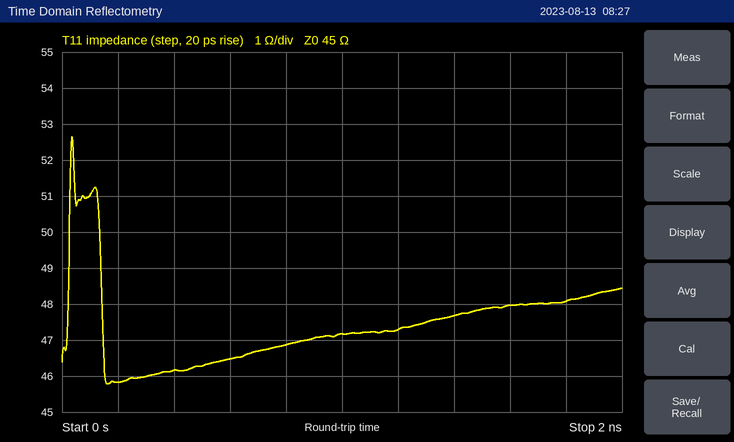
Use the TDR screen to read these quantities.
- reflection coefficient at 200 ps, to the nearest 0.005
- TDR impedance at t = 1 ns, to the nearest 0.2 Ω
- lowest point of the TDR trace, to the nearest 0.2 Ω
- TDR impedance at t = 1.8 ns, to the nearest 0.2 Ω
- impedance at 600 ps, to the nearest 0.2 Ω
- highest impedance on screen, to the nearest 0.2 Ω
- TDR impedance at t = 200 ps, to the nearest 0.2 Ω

+0.010
47.2 Ω
45.8 Ω
48.0 Ω
46.4 Ω
52.6 Ω
45.8 Ω
